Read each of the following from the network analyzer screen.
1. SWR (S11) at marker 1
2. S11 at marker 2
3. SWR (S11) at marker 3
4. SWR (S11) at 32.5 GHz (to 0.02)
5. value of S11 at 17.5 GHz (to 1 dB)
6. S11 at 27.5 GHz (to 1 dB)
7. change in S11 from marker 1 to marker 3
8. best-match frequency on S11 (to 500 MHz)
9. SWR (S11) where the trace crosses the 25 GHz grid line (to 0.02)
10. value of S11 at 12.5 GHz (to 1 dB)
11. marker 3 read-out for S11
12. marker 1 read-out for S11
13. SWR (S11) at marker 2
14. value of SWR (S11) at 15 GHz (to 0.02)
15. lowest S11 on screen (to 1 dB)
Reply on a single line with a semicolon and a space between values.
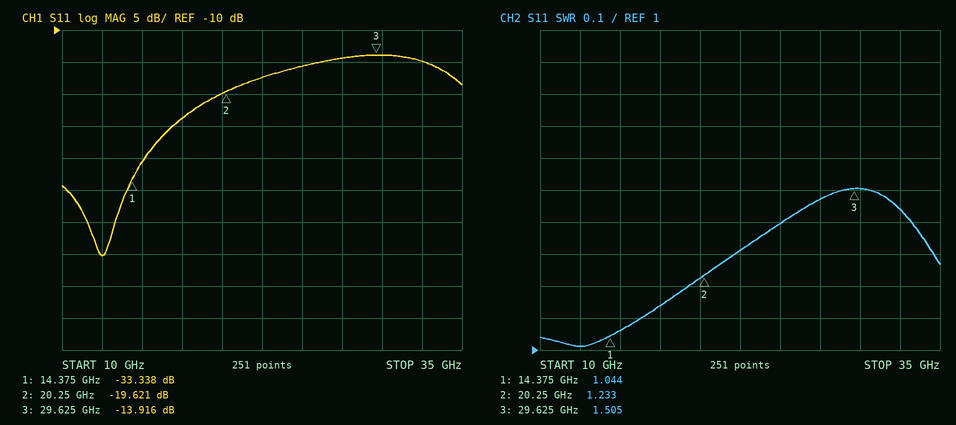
1.044; -19.621 dB; 1.505; 1.44; -24 dB; -14 dB; 19.422 dB; 12.5 GHz; 1.40; -45 dB; -13.916 dB; -33.338 dB; 1.233; 1.06; -45 dB
